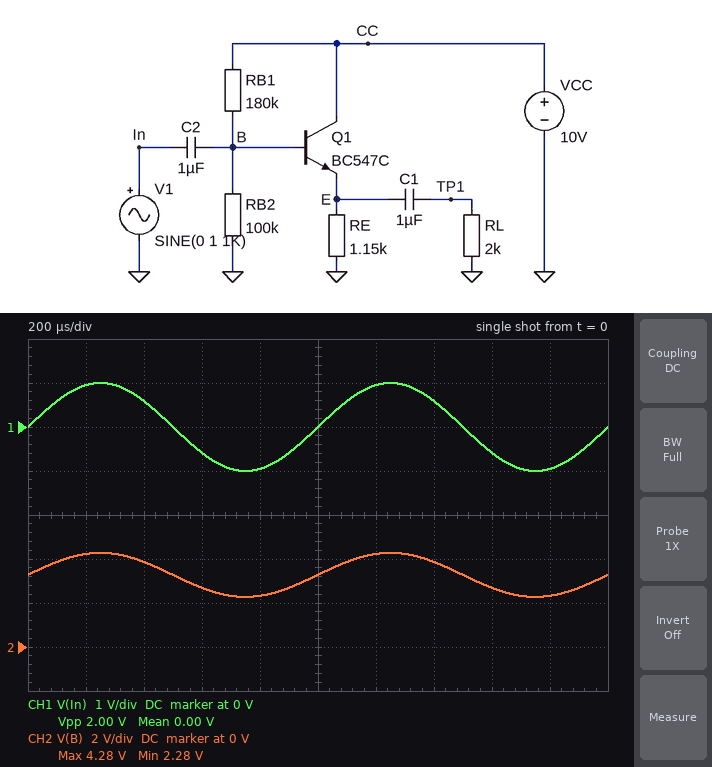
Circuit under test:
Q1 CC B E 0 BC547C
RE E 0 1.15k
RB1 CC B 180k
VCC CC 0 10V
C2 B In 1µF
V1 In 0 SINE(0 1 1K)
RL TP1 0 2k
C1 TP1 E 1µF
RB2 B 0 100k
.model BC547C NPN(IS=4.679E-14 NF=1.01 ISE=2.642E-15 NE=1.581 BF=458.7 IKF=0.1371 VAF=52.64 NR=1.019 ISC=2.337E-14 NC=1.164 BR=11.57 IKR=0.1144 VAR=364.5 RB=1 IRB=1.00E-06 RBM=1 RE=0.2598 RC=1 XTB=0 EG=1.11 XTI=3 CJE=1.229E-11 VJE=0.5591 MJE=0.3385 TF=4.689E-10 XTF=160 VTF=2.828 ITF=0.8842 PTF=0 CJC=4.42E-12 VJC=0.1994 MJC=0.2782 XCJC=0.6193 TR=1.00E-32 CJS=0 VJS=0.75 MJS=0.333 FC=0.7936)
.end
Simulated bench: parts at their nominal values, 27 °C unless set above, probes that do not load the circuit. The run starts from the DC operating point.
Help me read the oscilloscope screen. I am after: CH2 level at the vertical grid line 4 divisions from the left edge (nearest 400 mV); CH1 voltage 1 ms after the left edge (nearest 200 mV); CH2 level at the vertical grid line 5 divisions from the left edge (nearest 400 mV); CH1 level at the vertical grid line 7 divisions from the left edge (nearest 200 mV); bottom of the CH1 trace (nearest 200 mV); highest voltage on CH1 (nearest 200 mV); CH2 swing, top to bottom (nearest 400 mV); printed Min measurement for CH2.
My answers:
2.4 V
0 V
3.2 V
600 mV
-1.0 V
1.0 V
2.0 V
2.28 V
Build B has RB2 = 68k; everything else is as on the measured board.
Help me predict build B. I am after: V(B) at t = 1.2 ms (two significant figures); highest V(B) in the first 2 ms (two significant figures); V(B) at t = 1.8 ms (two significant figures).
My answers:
3.5 V
3.6 V
1.6 V
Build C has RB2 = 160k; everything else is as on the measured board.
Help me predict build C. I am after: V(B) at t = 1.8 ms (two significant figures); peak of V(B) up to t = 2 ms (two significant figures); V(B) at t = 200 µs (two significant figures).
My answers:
3.2 V
5.2 V
5.1 V
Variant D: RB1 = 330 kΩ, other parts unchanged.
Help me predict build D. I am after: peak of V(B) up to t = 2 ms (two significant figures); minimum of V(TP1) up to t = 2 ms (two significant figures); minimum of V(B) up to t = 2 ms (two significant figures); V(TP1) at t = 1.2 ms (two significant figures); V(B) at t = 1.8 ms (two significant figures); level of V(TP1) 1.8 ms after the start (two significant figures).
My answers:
3.1 V
-960 mV
1.1 V
900 mV
1.2 V
-890 mV
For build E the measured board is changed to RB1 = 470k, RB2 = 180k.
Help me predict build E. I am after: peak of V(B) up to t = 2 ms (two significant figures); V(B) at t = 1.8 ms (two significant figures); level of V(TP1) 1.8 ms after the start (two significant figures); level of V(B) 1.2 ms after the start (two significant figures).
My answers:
3.4 V
1.4 V
-910 mV
3.3 V
